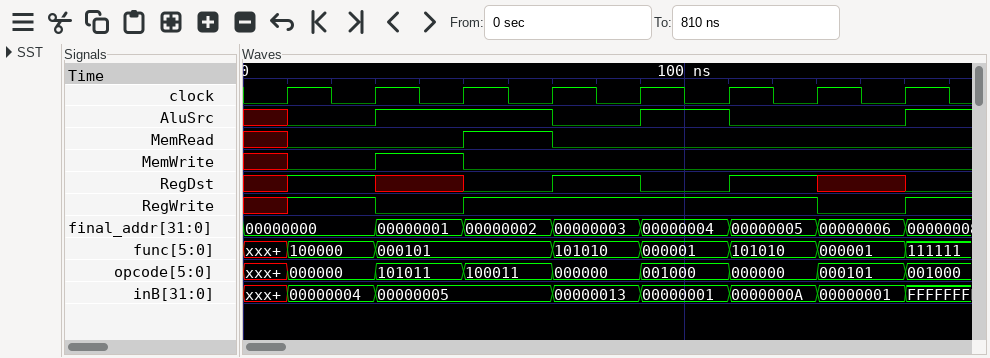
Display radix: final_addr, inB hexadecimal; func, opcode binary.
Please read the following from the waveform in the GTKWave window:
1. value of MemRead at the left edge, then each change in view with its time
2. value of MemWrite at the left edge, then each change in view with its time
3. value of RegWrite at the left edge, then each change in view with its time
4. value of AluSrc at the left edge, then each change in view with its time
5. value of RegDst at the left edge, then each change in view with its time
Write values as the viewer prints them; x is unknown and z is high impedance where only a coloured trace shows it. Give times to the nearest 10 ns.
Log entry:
x, 0 at 10 ns, 1 at 50 ns, 0 at 70 ns
x, 0 at 10 ns, 1 at 30 ns, 0 at 50 ns
x, 1 at 10 ns, 0 at 30 ns, 1 at 50 ns, 0 at 130 ns, 1 at 150 ns
x, 0 at 10 ns, 1 at 30 ns, 0 at 70 ns, 1 at 90 ns, 0 at 110 ns, 1 at 150 ns
x, 1 at 10 ns, x at 30 ns, 0 at 50 ns, 1 at 70 ns, 0 at 90 ns, 1 at 110 ns, x at 130 ns, 0 at 150 ns
